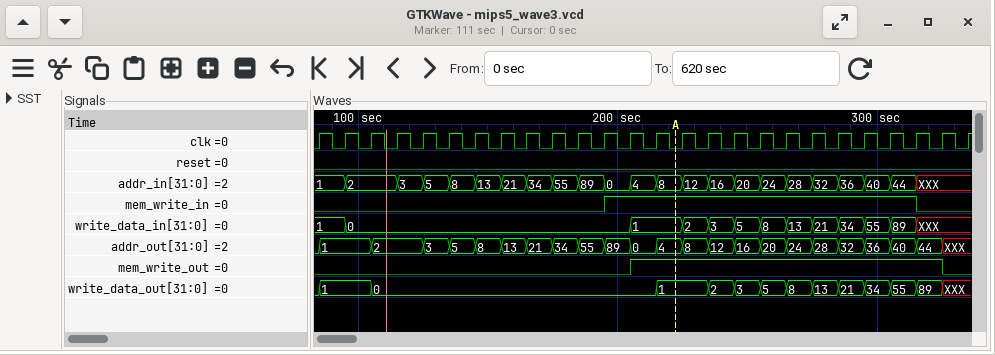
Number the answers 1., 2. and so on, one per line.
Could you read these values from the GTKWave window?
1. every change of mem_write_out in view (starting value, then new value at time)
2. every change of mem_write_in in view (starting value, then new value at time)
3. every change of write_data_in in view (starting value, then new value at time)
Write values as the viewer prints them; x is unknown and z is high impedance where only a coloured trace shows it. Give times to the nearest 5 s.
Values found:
1. 0, 1 at 205 s, 0 at 325 s
2. 0, 1 at 195 s, 0 at 315 s
3. 1, 0 at 95 s, 1 at 205 s, 2 at 225 s, 3 at 235 s, 5 at 245 s, 8 at 255 s, 13 at 265 s, 21 at 275 s, 34 at 285 s, 55 at 295 s, 89 at 305 s, XXX at 315 s
